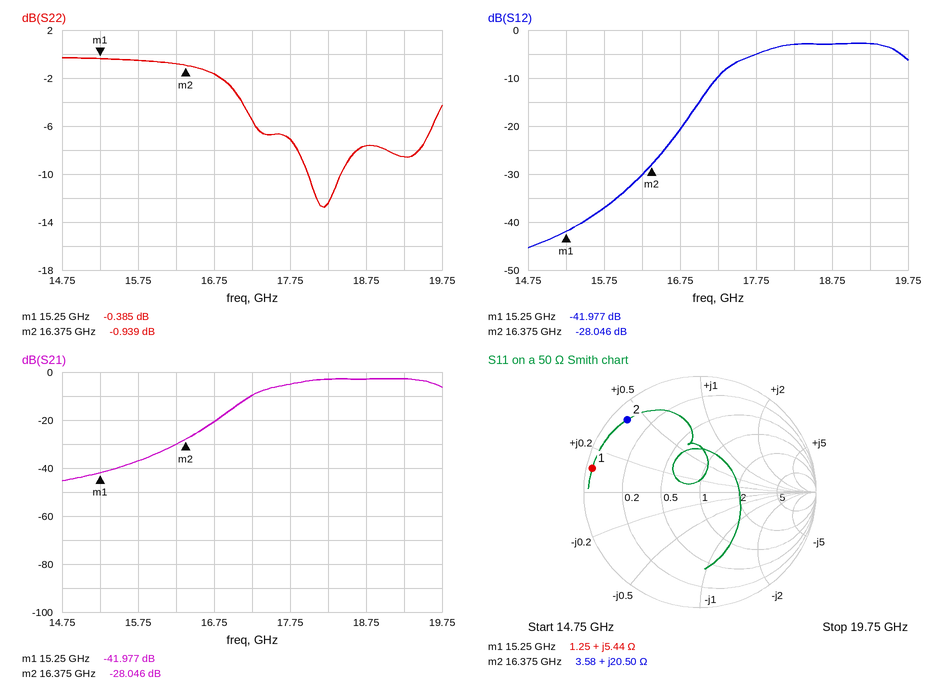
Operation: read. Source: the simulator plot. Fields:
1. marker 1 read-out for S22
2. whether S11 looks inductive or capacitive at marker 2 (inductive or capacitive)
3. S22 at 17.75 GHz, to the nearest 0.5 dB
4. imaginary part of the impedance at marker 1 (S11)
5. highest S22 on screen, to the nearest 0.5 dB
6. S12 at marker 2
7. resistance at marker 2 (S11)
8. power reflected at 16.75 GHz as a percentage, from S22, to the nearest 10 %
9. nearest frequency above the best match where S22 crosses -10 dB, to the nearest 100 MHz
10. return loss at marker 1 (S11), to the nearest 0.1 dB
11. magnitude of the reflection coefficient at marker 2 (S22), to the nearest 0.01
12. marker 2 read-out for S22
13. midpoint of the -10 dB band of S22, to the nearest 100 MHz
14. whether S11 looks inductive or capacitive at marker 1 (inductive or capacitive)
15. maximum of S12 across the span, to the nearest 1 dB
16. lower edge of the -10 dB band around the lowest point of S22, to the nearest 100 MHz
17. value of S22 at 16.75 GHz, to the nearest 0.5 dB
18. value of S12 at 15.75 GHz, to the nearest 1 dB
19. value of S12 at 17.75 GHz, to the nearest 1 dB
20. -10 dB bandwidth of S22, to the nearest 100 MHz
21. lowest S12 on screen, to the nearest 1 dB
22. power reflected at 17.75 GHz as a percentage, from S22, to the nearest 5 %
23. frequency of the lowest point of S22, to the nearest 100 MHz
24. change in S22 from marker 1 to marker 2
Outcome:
-0.385 dB
inductive
-7.0 dB
+5.44 Ω
-0.5 dB
-28.046 dB
3.58 Ω
70 %
18.4 GHz
0.4 dB
0.90
-0.939 dB
18.2 GHz
inductive
-3 dB
18.0 GHz
-1.5 dB
-37 dB
-5 dB
400 MHz
-45 dB
20 %
18.2 GHz
-0.554 dB
